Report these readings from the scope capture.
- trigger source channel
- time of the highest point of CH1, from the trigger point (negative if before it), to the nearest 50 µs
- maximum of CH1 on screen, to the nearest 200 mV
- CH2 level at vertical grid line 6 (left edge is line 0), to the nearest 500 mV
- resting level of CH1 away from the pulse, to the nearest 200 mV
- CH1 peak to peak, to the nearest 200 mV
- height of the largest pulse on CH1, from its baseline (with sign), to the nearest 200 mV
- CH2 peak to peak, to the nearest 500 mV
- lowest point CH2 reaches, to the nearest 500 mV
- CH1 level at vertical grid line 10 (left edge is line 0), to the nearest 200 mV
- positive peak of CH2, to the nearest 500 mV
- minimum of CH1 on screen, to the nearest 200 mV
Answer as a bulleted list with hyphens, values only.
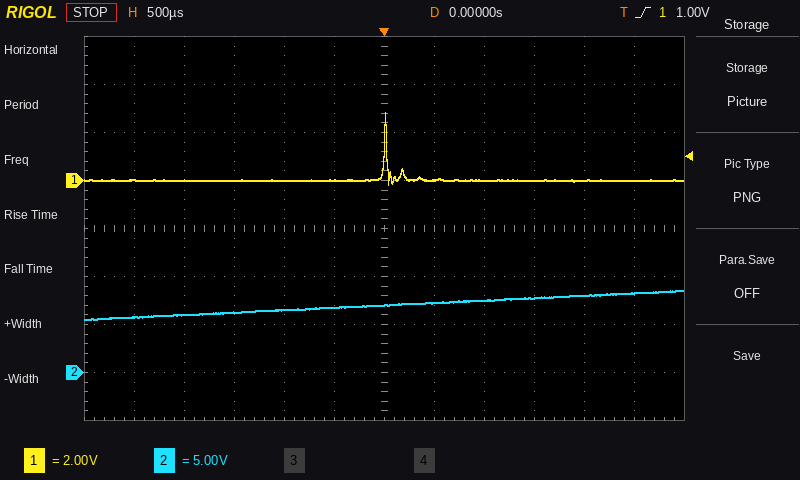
- CH1
- 0 µs
- 2.8 V
- 7.0 V
- 0.0 V
- 3.0 V
- +2.8 V
- 3.0 V
- 5.5 V
- 0.0 V
- 8.5 V
- -200 mV
